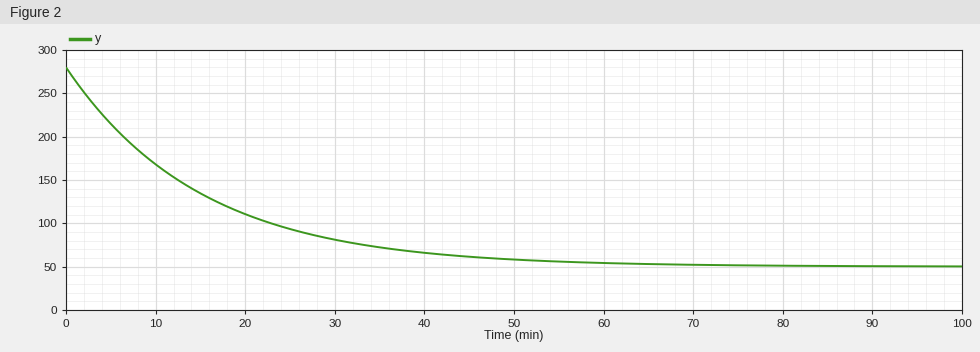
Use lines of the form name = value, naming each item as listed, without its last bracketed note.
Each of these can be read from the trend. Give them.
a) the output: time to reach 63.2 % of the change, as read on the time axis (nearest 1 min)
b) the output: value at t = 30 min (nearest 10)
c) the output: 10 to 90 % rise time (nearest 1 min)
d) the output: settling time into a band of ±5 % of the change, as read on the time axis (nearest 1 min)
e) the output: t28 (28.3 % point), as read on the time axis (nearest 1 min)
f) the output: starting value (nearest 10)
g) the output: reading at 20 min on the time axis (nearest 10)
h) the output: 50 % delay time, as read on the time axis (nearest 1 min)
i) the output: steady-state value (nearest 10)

the output: time to reach 63.2 % of the change, as read on the time axis = 15 min
the output: value at t = 30 min = 80
the output: 10 to 90 % rise time = 33 min
the output: settling time into a band of ±5 % of the change, as read on the time axis = 45 min
the output: t28 (28.3 % point), as read on the time axis = 5 min
the output: starting value = 280
the output: reading at 20 min on the time axis = 110
the output: 50 % delay time, as read on the time axis = 10 min
the output: steady-state value = 50
